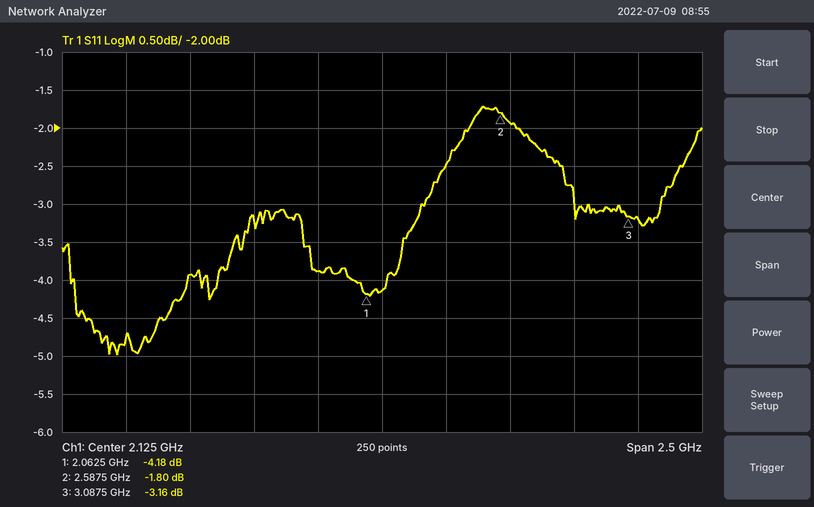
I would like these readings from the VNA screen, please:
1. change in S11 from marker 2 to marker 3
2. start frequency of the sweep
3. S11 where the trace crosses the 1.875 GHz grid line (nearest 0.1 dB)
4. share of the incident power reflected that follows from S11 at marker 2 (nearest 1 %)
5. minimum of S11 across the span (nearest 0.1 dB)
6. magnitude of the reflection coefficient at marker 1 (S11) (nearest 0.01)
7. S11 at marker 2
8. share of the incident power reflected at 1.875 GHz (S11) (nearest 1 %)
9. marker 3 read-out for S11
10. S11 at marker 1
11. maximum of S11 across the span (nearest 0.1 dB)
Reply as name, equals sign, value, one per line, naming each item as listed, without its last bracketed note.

change in S11 from marker 2 to marker 3 = -1.36 dB
start frequency of the sweep = 875 MHz
S11 where the trace crosses the 1.875 GHz grid line = -3.9 dB
share of the incident power reflected that follows from S11 at marker 2 = 66 %
minimum of S11 across the span = -5.0 dB
magnitude of the reflection coefficient at marker 1 (S11) = 0.62
S11 at marker 2 = -1.80 dB
share of the incident power reflected at 1.875 GHz (S11) = 41 %
marker 3 read-out for S11 = -3.16 dB
S11 at marker 1 = -4.18 dB
maximum of S11 across the span = -1.7 dB
